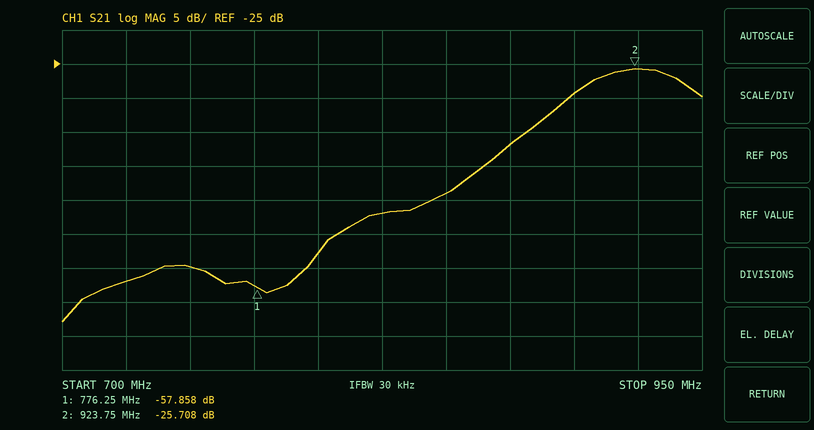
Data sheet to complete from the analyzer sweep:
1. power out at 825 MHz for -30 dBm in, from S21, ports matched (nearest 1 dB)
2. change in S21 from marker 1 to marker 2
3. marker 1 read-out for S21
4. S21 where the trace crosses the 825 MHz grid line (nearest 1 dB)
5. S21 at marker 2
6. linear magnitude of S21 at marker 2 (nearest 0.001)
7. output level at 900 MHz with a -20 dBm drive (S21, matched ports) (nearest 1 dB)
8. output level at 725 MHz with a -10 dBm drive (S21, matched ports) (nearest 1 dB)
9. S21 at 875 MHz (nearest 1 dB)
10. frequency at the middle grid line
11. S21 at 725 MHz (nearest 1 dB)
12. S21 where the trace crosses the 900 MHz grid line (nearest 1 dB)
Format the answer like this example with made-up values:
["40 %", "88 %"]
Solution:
["-77 dBm", "32.150 dB", "-57.858 dB", "-47 dB", "-25.708 dB", "0.052", "-49 dBm", "-67 dBm", "-37 dB", "825 MHz", "-57 dB", "-29 dB"]
